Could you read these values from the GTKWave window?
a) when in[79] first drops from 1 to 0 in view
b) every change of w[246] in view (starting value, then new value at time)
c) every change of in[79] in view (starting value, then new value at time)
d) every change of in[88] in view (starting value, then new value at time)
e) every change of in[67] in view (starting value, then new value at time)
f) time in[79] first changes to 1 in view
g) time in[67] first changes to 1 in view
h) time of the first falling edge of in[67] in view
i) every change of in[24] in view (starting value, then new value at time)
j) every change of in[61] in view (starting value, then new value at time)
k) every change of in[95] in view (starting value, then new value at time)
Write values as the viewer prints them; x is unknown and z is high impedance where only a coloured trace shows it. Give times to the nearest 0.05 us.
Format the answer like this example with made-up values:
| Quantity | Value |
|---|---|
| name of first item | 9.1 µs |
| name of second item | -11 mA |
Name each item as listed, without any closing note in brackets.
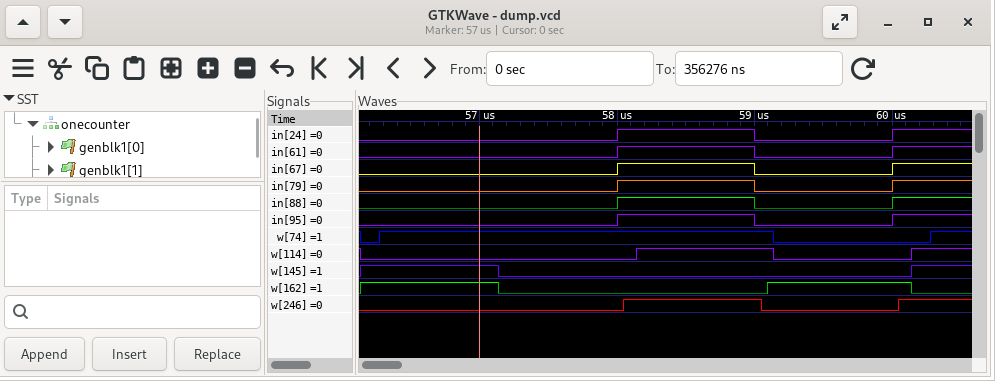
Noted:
| Quantity | Value |
|---|---|
| when in[79] first drops from 1 to 0 in view | 59 us |
| every change of w[246] in view | 0, 1 at 58.05 us, 0 at 59.05 us, 1 at 60.05 us |
| every change of in[79] in view | 0, 1 at 58 us, 0 at 59 us, 1 at 60 us |
| every change of in[88] in view | 0, 1 at 58 us, 0 at 59 us, 1 at 60 us |
| every change of in[67] in view | 0, 1 at 58 us, 0 at 59 us, 1 at 60 us |
| time in[79] first changes to 1 in view | 58 us |
| time in[67] first changes to 1 in view | 58 us |
| time of the first falling edge of in[67] in view | 59 us |
| every change of in[24] in view | 0, 1 at 58 us, 0 at 59 us, 1 at 60 us |
| every change of in[61] in view | 0, 1 at 58 us, 0 at 59 us, 1 at 60 us |
| every change of in[95] in view | 0, 1 at 58 us, 0 at 59 us, 1 at 60 us |
